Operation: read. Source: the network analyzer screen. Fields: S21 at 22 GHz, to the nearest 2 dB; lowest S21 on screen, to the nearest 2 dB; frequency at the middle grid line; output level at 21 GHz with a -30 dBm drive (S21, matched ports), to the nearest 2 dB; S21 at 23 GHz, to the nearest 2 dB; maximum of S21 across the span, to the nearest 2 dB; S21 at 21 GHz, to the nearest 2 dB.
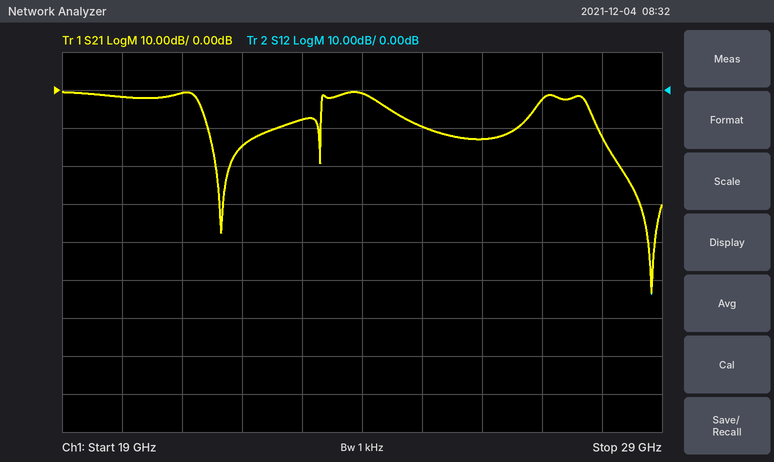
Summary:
-14 dB
-54 dB
24 GHz
-30 dBm
-8 dB
0 dB
0 dB
